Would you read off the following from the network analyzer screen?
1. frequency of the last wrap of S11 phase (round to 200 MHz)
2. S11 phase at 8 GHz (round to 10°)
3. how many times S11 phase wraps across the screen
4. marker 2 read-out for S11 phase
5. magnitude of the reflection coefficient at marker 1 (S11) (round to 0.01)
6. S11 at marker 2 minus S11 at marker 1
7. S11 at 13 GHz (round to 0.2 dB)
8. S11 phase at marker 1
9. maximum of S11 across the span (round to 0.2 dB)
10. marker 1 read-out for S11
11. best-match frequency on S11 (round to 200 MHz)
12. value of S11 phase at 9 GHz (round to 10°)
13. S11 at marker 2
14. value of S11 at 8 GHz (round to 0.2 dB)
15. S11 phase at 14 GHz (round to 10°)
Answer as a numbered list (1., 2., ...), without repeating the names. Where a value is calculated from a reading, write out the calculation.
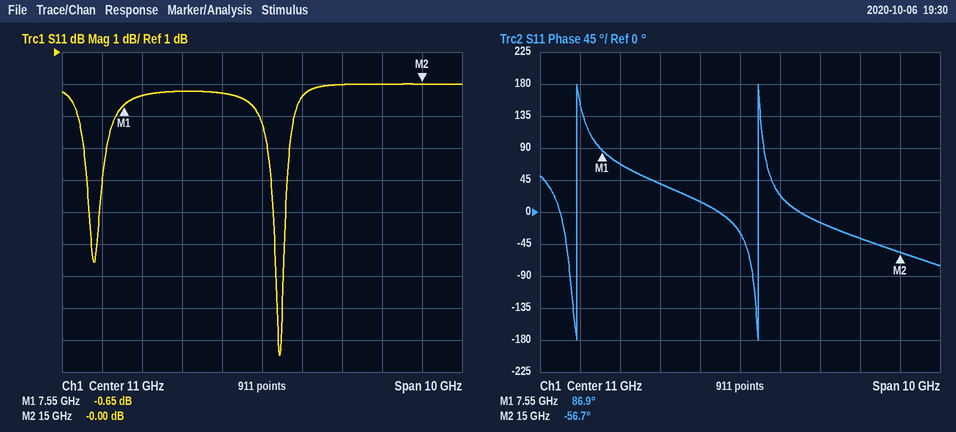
1. 11.4 GHz
2. 70°
3. 2
4. -56.7°
5. 10^(-0.65/20) ≈ 0.93
6. -0 − (-0.65) = 0.65 dB
7. 0.0 dB
8. 86.9°
9. 0.0 dB
10. -0.65 dB
11. 11.4 GHz
12. 40°
13. -0.00 dB
14. -0.4 dB
15. -40°
